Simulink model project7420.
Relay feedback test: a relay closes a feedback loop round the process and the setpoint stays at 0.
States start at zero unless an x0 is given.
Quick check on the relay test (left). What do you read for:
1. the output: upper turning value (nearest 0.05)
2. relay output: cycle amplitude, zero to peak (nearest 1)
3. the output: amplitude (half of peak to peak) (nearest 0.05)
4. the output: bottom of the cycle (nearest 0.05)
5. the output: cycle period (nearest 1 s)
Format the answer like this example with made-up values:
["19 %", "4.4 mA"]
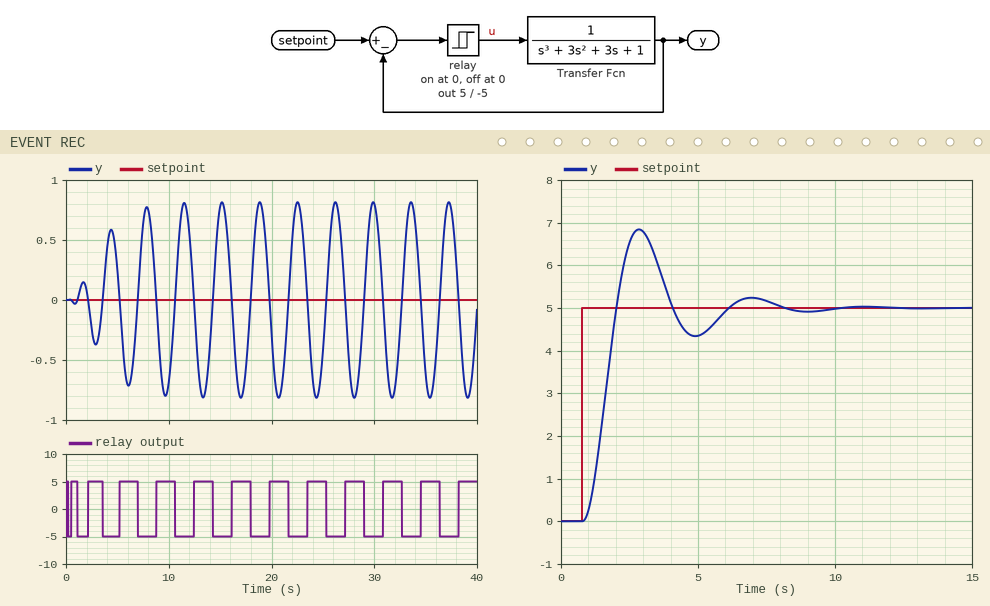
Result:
["0.80", "5", "0.80", "-0.80", "4 s"]
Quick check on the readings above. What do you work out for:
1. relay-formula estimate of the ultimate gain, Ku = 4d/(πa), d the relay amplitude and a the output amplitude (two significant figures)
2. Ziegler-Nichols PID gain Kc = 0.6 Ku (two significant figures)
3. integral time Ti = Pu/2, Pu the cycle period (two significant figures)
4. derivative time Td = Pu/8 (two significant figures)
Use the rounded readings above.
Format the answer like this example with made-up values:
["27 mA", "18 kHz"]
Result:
["8.0", "4.8", "2.0 s", "0.50 s"]
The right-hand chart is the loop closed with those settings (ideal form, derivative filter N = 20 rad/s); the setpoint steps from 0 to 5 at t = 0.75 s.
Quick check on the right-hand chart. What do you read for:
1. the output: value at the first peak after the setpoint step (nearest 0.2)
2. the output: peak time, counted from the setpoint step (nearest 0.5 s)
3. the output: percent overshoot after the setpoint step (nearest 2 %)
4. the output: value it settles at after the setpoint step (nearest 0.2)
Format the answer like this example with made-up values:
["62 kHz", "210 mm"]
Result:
["6.8", "2.0 s", "36 %", "5.0"]
